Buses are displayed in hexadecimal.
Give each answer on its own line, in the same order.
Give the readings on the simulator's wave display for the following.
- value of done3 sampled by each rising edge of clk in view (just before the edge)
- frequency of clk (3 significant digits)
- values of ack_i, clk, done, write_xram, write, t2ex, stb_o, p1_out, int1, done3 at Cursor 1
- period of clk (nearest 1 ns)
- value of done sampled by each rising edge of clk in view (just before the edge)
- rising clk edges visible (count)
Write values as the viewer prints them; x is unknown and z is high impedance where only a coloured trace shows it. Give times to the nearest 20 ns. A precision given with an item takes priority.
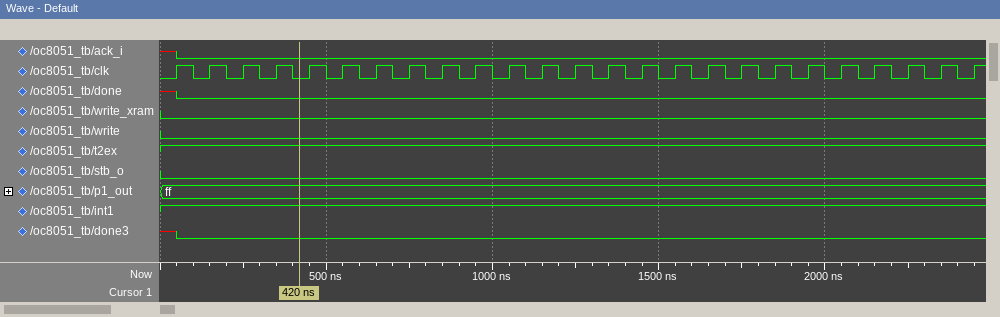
x 0 0 0 0 0 0 0 0 0 0 0 0 0 0 0 0 0 0 0 0 0 0 0 0
10.0 MHz
ack_i=0, clk=0, done=0, write_xram=0, write=0, t2ex=1, stb_o=0, p1_out=ff, int1=1, done3=0
100 ns
x 0 0 0 0 0 0 0 0 0 0 0 0 0 0 0 0 0 0 0 0 0 0 0 0
25
